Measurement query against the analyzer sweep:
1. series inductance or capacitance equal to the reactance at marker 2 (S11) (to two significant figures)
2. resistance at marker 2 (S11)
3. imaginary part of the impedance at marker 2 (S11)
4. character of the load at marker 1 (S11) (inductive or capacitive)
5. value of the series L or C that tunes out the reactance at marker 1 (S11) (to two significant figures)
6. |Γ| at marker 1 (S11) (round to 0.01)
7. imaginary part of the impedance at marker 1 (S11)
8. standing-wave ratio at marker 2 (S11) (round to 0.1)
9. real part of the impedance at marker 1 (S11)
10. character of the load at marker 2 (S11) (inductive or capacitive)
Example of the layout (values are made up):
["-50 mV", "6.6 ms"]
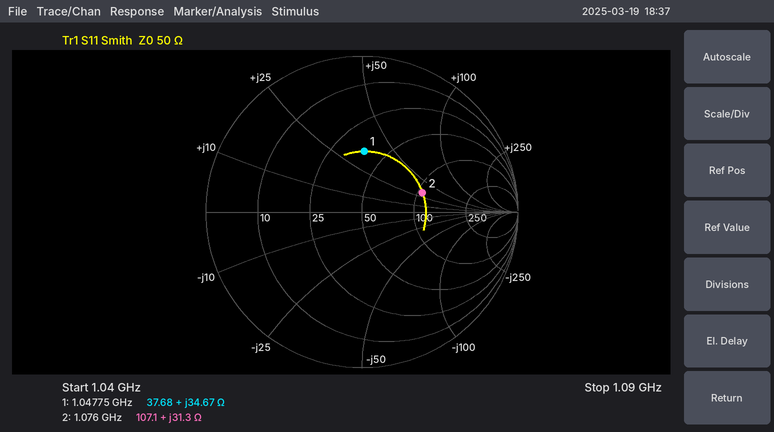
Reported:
["4.6 nH", "107.1 Ω", "+31.3 Ω", "inductive", "4.4 pF", "0.39", "+34.67 Ω", "2.4", "37.68 Ω", "inductive"]
